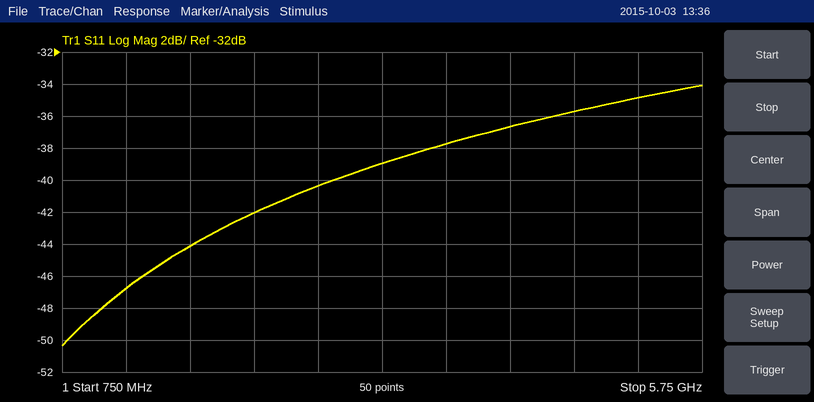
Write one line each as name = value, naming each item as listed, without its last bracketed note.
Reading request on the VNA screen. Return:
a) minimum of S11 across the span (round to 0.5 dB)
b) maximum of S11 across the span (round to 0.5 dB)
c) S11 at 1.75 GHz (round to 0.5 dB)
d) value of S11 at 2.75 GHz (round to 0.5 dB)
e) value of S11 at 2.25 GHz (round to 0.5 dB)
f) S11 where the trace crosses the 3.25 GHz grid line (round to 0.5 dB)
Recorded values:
minimum of S11 across the span = -50.5 dB
maximum of S11 across the span = -34.0 dB
S11 at 1.75 GHz = -44.0 dB
value of S11 at 2.75 GHz = -40.5 dB
value of S11 at 2.25 GHz = -42.0 dB
S11 where the trace crosses the 3.25 GHz grid line = -39.0 dB
